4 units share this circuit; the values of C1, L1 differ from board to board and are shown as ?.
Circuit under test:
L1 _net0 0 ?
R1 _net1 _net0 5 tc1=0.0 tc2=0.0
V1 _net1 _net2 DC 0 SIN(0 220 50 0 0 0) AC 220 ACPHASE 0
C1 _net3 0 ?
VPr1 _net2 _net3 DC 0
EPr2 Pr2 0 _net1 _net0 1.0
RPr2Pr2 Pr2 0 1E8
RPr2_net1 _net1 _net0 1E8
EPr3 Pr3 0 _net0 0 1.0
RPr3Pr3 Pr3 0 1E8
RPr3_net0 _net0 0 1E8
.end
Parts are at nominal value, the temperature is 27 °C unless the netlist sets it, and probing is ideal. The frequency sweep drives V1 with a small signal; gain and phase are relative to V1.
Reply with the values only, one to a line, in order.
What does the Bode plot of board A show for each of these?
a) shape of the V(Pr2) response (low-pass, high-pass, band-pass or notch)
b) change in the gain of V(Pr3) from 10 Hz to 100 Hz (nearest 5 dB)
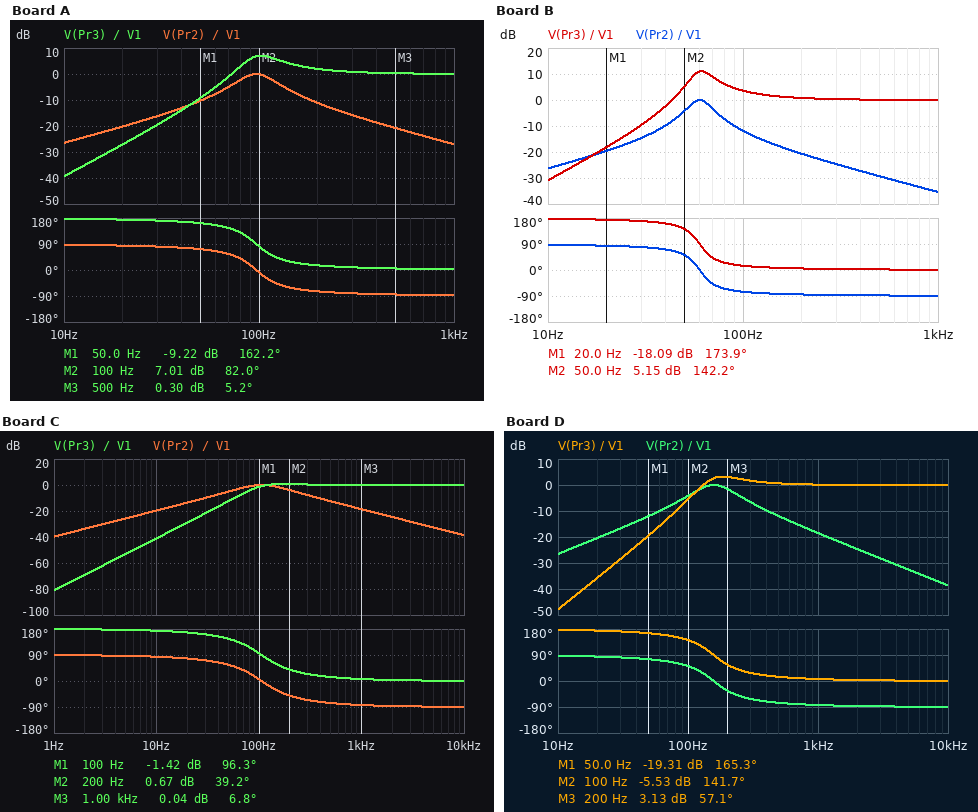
band-pass
45 dB
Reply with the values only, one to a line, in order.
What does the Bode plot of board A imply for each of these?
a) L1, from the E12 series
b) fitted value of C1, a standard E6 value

18 mH
150 µF
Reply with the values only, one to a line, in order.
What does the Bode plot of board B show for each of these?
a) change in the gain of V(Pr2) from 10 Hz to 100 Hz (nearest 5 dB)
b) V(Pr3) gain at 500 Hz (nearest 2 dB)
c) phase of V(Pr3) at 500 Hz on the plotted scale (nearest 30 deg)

15 dB
0 dB
0 deg
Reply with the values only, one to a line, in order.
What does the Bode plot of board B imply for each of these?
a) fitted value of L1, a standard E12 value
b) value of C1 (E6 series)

47 mH
150 µF
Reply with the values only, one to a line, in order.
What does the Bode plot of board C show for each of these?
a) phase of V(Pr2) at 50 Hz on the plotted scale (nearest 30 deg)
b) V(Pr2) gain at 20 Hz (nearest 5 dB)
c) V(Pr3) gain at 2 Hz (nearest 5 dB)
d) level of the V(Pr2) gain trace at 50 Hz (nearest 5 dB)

60 deg
-15 dB
-70 dB
-5 dB
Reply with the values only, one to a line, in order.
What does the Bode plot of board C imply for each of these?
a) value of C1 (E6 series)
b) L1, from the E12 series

330 µF
6.8 mH
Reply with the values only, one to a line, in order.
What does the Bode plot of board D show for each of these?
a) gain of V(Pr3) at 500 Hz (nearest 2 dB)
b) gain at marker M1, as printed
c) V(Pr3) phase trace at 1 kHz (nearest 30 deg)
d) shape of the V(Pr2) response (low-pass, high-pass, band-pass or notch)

0 dB
-19.31 dB
0 deg
band-pass
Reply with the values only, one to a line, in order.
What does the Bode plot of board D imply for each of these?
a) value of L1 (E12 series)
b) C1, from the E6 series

6.8 mH
150 µF
